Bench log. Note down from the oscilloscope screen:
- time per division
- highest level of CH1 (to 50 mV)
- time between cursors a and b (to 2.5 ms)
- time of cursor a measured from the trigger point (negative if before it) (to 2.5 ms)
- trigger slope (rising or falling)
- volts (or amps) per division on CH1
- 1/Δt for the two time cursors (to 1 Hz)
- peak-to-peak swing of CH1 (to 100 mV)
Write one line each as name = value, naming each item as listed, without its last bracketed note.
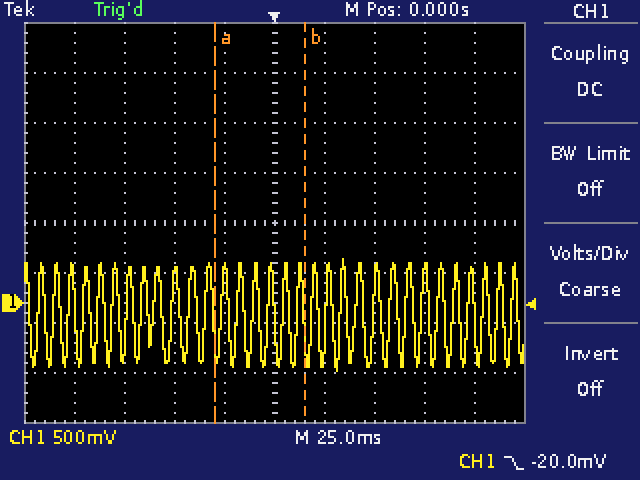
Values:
time per division = 25 ms
highest level of CH1 = 450 mV
time between cursors a and b = 45.0 ms
time of cursor a measured from the trigger point (negative if before it) = -30.0 ms
trigger slope = falling
volts (or amps) per division on CH1 = 500 mV
1/Δt for the two time cursors = 22 Hz
peak-to-peak swing of CH1 = 1.10 V
